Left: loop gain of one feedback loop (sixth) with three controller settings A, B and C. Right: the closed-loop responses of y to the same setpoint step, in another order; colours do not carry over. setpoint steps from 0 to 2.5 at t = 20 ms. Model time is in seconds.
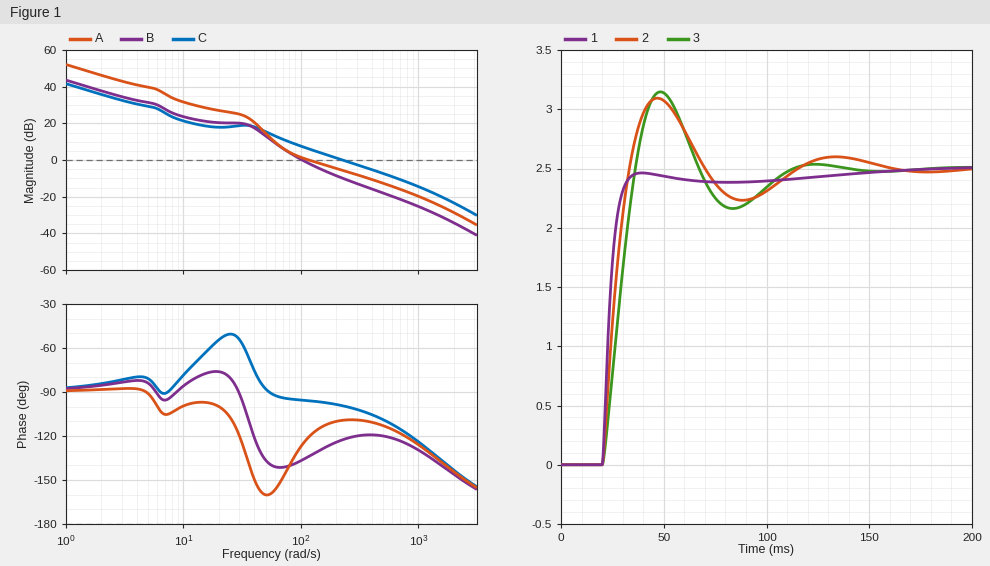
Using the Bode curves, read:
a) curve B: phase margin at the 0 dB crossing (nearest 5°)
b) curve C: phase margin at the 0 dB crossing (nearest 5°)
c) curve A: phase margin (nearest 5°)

45°
80°
60°
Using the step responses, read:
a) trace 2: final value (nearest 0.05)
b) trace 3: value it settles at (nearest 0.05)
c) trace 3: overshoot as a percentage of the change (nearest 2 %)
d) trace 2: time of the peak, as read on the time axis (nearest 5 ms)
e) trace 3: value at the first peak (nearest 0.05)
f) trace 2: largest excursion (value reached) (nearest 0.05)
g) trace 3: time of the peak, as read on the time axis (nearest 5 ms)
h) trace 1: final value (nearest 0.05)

2.50
2.50
26 %
45 ms
3.15
3.10
50 ms
2.50
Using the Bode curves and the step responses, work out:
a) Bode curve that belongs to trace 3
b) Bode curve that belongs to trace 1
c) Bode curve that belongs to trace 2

B
C
A
